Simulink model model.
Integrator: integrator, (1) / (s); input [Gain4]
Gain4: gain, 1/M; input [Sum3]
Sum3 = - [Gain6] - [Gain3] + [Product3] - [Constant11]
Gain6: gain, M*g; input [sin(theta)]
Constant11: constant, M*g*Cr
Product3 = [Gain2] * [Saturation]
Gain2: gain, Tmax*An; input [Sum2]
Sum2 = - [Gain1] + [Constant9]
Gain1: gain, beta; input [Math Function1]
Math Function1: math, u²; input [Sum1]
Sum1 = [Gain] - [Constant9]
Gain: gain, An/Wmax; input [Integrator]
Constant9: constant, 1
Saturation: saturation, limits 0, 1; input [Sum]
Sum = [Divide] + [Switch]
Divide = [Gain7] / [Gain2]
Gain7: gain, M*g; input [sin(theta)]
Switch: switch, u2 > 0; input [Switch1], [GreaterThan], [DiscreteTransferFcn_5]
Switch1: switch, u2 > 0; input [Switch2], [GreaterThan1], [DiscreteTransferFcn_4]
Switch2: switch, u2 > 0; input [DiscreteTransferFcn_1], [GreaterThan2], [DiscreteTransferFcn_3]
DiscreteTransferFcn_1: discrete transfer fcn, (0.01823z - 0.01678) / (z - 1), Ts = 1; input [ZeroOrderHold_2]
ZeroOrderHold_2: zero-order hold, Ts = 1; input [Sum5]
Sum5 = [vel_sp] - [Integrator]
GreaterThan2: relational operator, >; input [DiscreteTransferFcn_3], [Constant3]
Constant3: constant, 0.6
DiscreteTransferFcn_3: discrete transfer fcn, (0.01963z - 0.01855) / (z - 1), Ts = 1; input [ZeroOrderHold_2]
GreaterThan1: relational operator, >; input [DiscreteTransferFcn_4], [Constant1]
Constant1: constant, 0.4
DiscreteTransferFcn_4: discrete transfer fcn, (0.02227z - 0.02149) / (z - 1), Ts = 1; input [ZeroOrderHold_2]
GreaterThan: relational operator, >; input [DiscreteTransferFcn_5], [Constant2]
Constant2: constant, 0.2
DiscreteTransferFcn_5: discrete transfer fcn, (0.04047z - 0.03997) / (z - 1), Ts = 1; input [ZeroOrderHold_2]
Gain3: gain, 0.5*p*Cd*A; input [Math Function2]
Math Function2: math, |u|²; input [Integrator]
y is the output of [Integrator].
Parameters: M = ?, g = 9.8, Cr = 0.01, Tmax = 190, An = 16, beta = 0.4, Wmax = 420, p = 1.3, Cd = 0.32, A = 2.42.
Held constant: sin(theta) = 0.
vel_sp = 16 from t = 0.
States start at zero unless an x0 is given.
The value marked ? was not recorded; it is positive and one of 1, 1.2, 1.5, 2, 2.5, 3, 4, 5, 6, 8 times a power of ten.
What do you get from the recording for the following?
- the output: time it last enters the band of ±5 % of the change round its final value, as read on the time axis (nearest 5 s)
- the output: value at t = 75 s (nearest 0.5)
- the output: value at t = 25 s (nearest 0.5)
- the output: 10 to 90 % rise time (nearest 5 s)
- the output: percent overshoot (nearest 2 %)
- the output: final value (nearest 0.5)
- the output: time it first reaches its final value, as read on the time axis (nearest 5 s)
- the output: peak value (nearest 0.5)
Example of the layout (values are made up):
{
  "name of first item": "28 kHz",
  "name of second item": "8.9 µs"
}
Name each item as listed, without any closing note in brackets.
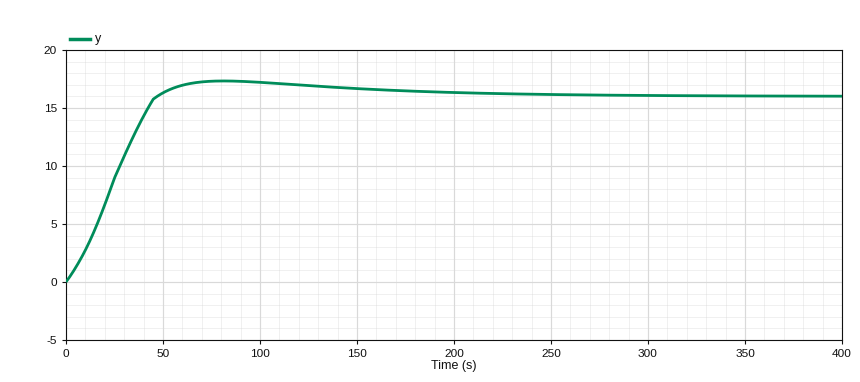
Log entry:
{
  "the output: time it last enters the band of ±5 % of the change round its final value, as read on the time axis": "135 s",
  "the output: value at t = 75 s": "17.5",
  "the output: value at t = 25 s": "9.0",
  "the output: 10 to 90 % rise time": "35 s",
  "the output: percent overshoot": "8 %",
  "the output: final value": "16.0",
  "the output: time it first reaches its final value, as read on the time axis": "45 s",
  "the output: peak value": "17.5"
}
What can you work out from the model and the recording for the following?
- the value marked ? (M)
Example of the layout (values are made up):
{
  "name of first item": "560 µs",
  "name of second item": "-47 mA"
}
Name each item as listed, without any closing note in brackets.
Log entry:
{
  "the value marked ?": "2000"
}
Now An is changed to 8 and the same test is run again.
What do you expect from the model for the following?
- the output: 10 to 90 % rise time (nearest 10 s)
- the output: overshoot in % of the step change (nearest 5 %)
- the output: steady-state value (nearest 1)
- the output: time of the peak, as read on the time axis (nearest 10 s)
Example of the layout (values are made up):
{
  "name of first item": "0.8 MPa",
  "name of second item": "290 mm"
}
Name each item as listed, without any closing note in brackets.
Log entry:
{
  "the output: 10 to 90 % rise time": "40 s",
  "the output: overshoot in % of the step change": "15 %",
  "the output: steady-state value": "16",
  "the output: time of the peak, as read on the time axis": "70 s"
}
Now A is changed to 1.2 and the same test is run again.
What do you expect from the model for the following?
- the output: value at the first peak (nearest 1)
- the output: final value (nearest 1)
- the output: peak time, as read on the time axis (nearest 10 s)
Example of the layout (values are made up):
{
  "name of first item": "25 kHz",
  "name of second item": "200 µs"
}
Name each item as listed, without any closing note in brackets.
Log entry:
{
  "the output: value at the first peak": "18",
  "the output: final value": "16",
  "the output: peak time, as read on the time axis": "80 s"
}
